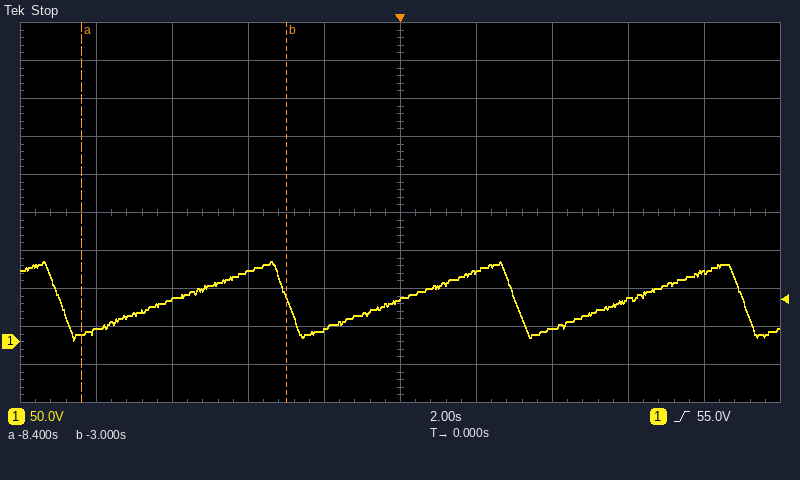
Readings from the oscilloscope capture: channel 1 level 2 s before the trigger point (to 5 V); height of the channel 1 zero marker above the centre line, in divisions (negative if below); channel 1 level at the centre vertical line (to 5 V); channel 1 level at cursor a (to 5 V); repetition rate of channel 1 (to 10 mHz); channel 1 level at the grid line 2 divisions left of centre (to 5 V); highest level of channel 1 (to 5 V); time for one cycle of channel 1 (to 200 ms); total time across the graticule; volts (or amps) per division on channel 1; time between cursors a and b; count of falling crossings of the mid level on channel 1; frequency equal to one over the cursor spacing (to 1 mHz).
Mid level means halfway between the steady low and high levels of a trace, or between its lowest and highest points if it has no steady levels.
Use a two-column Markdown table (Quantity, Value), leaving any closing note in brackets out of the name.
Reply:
| Quantity | Value |
|---|---|
| channel 1 level 2 s before the trigger point | 15 V |
| height of the channel 1 zero marker above the centre line, in divisions | -3.4 div |
| channel 1 level at the centre vertical line | 55 V |
| channel 1 level at cursor a | 10 V |
| repetition rate of channel 1 | 170 mHz |
| channel 1 level at the grid line 2 divisions left of centre | 90 V |
| highest level of channel 1 | 105 V |
| time for one cycle of channel 1 | 6.0 s |
| total time across the graticule | 20 s |
| volts (or amps) per division on channel 1 | 50 V |
| time between cursors a and b | 5.4 s |
| count of falling crossings of the mid level on channel 1 | 4 |
| frequency equal to one over the cursor spacing | 185 mHz |
